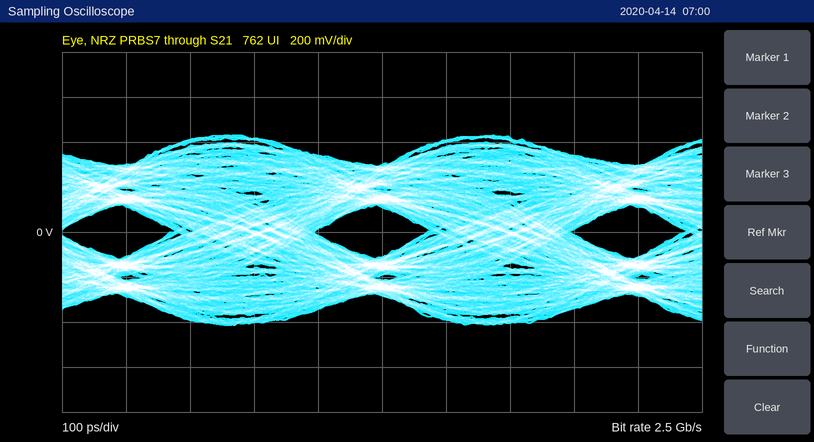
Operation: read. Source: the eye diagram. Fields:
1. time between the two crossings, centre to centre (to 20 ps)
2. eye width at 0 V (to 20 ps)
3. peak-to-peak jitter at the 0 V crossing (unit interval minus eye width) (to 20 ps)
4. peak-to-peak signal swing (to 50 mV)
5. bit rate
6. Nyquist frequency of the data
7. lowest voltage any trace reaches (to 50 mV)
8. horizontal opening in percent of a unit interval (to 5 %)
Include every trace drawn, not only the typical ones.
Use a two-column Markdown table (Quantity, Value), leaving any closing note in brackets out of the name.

| Quantity | Value |
|---|---|
| time between the two crossings, centre to centre | 400 ps |
| eye width at 0 V | 180 ps |
| peak-to-peak jitter at the 0 V crossing (unit interval minus eye width) | 220 ps |
| peak-to-peak signal swing | 850 mV |
| bit rate | 2.5 Gb/s |
| Nyquist frequency of the data | 1.25 GHz |
| lowest voltage any trace reaches | -400 mV |
| horizontal opening in percent of a unit interval | 45 % |
